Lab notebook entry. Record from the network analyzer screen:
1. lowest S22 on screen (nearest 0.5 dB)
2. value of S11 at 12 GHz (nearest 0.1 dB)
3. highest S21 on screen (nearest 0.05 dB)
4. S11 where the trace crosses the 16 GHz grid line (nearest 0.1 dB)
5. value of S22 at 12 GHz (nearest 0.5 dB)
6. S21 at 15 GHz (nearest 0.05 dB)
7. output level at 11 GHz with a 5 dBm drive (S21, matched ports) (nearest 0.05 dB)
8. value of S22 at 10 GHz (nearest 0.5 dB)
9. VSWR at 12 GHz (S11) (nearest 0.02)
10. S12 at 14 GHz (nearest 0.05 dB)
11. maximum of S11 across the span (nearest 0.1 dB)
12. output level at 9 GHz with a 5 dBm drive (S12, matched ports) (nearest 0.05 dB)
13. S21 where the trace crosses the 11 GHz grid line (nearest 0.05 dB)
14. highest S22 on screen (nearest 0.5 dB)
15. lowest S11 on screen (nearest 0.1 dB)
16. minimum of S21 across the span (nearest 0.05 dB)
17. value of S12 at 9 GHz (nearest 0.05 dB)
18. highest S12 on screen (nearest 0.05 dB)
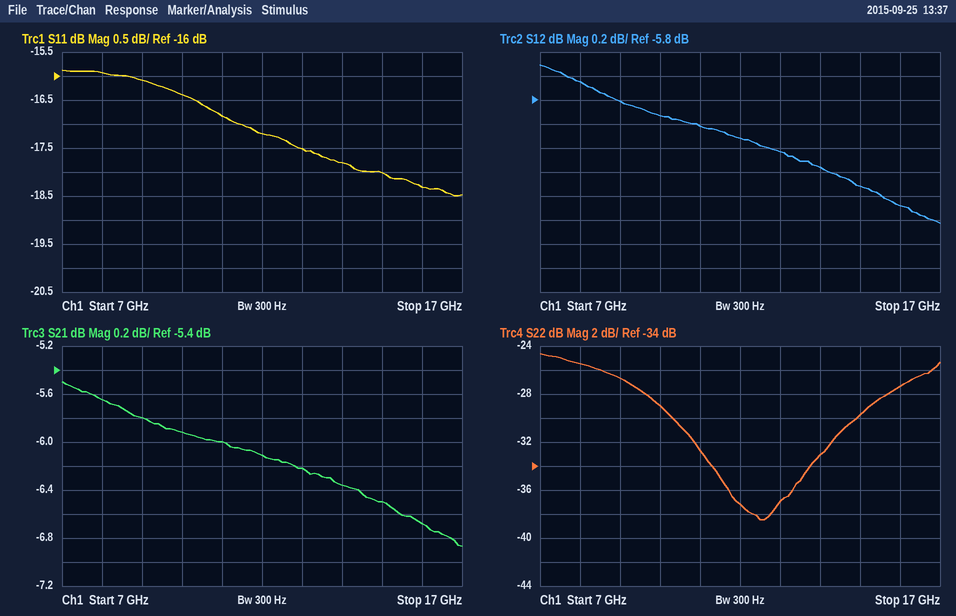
-38.5 dB
-17.2 dB
-5.50 dB
-18.3 dB
-37.0 dB
-6.50 dB
-1.00 dBm
-29.0 dB
1.32
-6.35 dB
-15.9 dB
-0.80 dBm
-6.00 dB
-24.5 dB
-18.5 dB
-6.85 dB
-5.80 dB
-5.50 dB
